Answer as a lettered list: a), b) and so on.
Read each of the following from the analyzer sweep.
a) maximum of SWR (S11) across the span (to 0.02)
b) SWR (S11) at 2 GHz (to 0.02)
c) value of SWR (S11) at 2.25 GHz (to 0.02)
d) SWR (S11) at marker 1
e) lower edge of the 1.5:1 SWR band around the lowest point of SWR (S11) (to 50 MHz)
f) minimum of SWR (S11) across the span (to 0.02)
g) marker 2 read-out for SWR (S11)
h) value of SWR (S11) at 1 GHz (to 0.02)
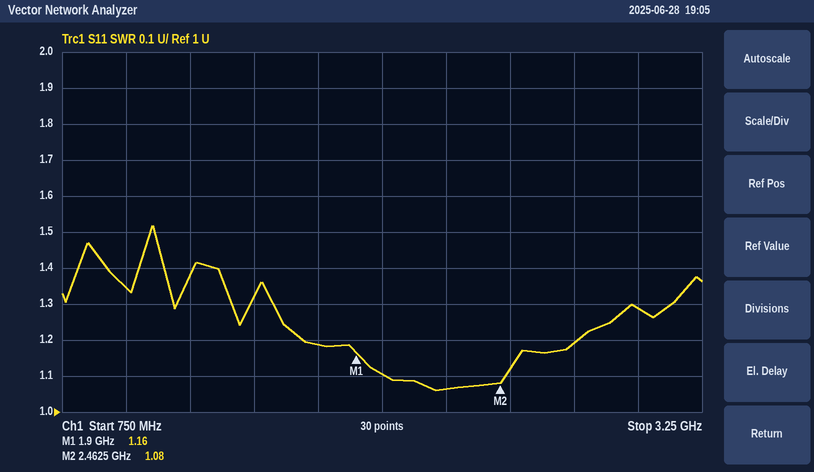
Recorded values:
a) 1.52
b) 1.10
c) 1.06
d) 1.16
e) 1.10 GHz
f) 1.06
g) 1.08
h) 1.34
